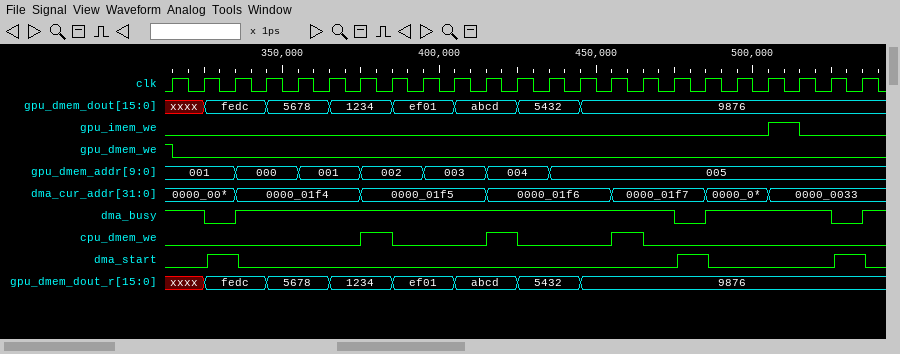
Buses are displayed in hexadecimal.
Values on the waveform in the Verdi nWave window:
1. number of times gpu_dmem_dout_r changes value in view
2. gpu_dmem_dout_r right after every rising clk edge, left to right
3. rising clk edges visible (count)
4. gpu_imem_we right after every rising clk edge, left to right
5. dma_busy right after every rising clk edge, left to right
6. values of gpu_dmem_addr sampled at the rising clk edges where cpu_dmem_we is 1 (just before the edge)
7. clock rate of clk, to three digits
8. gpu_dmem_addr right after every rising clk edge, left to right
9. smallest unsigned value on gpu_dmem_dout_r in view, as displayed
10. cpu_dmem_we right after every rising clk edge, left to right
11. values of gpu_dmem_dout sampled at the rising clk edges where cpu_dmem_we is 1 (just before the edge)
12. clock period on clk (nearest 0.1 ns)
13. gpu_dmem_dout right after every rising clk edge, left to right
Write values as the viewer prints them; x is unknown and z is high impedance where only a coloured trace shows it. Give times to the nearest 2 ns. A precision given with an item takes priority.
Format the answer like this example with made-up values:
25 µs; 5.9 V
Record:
7; xxxx, fedc, fedc, 5678, 5678, 1234, 1234, ef01, ef01, abcd, abcd, 5432, 5432, 9876, 9876, 9876, 9876, 9876, 9876, 9876, 9876, 9876, 9876; 23; 0 0 0 0 0 0 0 0 0 0 0 0 0 0 0 0 0 0 0 1 0 0 0; 1 0 1 1 1 1 1 1 1 1 1 1 1 1 1 1 0 1 1 1 1 0 1; 002, 004, 005; 100 MHz; 001, 001, 000, 000, 001, 001, 002, 002, 003, 003, 004, 004, 005, 005, 005, 005, 005, 005, 005, 005, 005, 005, 005; 1234; 0 0 0 0 0 0 1 0 0 0 1 0 0 0 1 0 0 0 0 0 0 0 0; 1234, abcd, 9876; 10 ns; xxxx, fedc, fedc, 5678, 5678, 1234, 1234, ef01, ef01, abcd, abcd, 5432, 5432, 9876, 9876, 9876, 9876, 9876, 9876, 9876, 9876, 9876, 9876
